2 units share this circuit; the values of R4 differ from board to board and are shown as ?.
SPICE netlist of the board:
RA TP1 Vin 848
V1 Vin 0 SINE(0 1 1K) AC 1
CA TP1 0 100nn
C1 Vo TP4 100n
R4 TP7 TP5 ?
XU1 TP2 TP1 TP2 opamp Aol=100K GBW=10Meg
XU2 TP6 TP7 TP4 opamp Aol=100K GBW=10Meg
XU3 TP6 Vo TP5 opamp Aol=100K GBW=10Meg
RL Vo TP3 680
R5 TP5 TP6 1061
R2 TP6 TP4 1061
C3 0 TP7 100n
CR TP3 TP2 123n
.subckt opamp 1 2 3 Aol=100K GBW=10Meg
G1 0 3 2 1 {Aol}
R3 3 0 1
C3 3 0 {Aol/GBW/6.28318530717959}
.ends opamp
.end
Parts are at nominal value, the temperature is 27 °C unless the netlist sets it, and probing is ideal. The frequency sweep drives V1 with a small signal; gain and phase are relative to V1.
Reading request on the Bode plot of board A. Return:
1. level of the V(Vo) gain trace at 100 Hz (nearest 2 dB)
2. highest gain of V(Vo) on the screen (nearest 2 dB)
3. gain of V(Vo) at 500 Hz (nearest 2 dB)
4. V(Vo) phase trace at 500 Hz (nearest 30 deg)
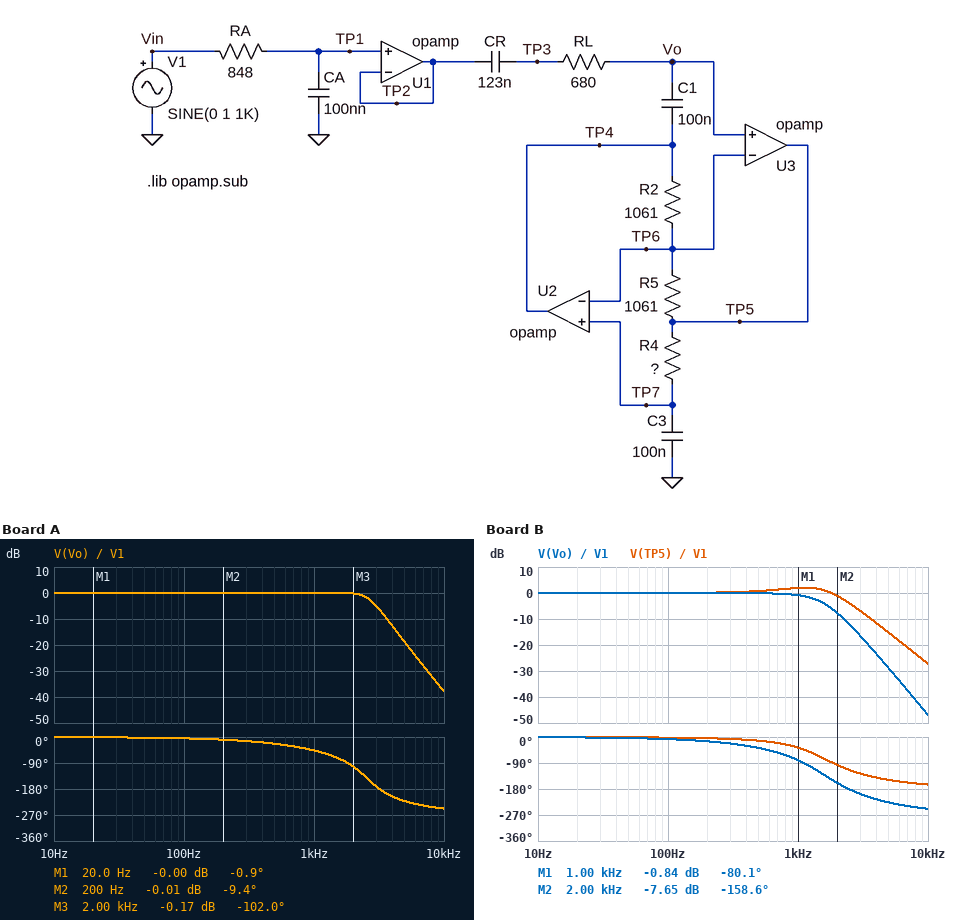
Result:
0 dB
0 dB
0 dB
-30 deg
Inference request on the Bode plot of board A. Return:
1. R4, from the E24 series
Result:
560 Ω
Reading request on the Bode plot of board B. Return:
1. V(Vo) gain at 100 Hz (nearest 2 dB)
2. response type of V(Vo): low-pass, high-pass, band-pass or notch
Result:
0 dB
low-pass
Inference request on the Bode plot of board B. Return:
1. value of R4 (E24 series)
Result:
1.5 kΩ
